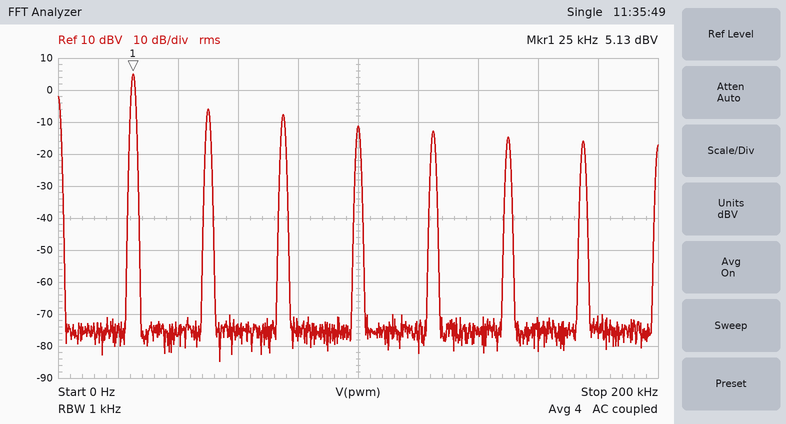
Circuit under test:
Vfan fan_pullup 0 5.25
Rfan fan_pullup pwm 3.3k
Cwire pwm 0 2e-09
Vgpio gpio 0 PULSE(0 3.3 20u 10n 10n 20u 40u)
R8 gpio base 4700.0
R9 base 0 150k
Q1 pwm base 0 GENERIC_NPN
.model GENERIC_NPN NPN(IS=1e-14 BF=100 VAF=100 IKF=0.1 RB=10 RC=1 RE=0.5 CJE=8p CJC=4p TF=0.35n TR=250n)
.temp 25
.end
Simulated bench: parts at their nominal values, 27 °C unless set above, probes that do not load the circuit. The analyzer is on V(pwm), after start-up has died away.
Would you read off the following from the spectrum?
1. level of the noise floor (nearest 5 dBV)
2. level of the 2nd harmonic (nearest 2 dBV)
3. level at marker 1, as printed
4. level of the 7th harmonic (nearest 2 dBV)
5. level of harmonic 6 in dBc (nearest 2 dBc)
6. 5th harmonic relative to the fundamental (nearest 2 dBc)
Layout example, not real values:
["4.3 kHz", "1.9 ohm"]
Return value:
["-75 dBV", "-6 dBV", "5.13 dBV", "-16 dBV", "-20 dBc", "-18 dBc"]
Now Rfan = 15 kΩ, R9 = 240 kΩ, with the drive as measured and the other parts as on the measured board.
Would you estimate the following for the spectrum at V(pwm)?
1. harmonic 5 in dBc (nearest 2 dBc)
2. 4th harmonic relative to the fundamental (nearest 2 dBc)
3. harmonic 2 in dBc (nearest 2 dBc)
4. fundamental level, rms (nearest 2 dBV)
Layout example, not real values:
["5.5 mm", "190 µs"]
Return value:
["-16 dBc", "-14 dBc", "-8 dBc", "-2 dBV"]
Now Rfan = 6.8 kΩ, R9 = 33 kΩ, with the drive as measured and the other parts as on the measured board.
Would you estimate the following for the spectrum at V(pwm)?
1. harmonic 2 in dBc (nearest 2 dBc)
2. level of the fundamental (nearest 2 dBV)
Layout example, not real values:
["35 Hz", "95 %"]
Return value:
["-10 dBc", "2 dBV"]
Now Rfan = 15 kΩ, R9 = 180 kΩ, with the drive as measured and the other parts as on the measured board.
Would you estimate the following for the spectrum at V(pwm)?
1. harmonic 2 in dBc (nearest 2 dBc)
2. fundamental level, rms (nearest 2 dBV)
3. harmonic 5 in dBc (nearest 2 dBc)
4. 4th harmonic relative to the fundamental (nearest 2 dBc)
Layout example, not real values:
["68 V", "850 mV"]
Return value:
["-8 dBc", "-2 dBV", "-16 dBc", "-14 dBc"]
